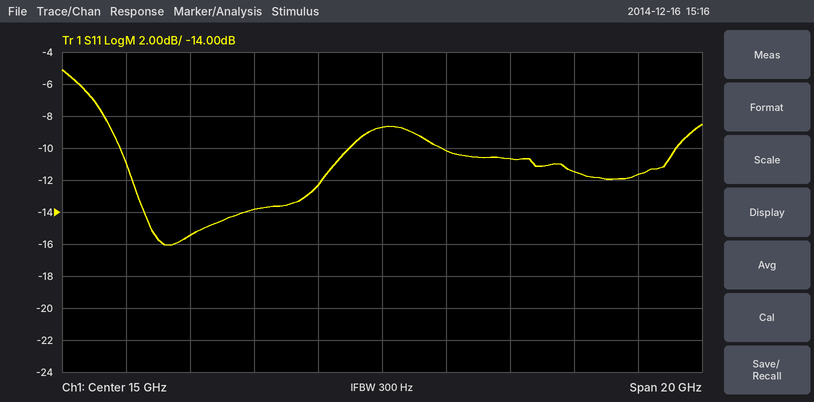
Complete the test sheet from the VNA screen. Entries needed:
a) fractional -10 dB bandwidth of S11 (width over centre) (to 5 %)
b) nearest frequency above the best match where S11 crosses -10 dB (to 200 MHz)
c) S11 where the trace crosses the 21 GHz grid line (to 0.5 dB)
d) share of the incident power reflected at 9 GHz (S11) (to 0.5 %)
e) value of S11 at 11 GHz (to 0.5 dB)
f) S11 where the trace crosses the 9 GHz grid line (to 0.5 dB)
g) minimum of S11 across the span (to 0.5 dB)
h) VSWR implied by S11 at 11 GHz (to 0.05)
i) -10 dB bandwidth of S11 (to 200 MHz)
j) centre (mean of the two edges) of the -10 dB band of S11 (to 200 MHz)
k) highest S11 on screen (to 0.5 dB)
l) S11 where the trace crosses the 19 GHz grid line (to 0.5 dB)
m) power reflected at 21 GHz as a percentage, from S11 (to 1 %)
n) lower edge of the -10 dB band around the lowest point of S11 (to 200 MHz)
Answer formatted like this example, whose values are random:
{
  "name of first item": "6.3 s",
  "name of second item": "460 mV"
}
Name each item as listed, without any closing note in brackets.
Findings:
{
  "fractional -10 dB bandwidth of S11 (width over centre)": "70 %",
  "nearest frequency above the best match where S11 crosses -10 dB": "14.0 GHz",
  "S11 where the trace crosses the 21 GHz grid line": "-11.5 dB",
  "share of the incident power reflected at 9 GHz (S11)": "3.0 %",
  "value of S11 at 11 GHz": "-14.0 dB",
  "S11 where the trace crosses the 9 GHz grid line": "-15.5 dB",
  "minimum of S11 across the span": "-16.0 dB",
  "VSWR implied by S11 at 11 GHz": "1.50",
  "-10 dB bandwidth of S11": "7.2 GHz",
  "centre (mean of the two edges) of the -10 dB band of S11": "10.4 GHz",
  "highest S11 on screen": "-5.0 dB",
  "S11 where the trace crosses the 19 GHz grid line": "-10.5 dB",
  "power reflected at 21 GHz as a percentage, from S11": "7 %",
  "lower edge of the -10 dB band around the lowest point of S11": "6.8 GHz"
}
